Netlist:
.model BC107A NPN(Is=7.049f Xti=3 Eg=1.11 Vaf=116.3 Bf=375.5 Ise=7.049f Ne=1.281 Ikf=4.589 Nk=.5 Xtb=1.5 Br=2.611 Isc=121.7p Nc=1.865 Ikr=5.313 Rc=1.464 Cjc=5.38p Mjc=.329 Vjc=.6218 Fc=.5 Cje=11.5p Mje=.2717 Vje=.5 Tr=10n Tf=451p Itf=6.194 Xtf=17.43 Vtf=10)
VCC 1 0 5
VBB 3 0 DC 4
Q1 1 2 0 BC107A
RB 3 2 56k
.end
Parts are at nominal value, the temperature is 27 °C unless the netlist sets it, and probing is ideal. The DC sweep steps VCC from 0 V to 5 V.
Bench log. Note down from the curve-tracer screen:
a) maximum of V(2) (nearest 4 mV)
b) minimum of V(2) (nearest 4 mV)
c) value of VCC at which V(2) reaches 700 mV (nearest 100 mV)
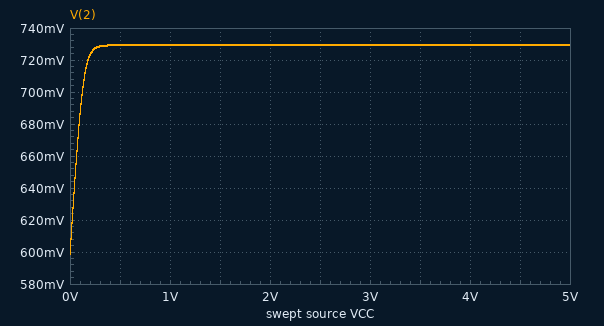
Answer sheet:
728 mV
600 mV
100 mV
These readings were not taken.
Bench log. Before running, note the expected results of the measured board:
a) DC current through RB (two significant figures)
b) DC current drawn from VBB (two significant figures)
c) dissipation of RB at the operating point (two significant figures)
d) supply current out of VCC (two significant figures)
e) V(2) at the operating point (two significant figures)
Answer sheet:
58 µA
58 µA
190 µW
13 mA
730 mV
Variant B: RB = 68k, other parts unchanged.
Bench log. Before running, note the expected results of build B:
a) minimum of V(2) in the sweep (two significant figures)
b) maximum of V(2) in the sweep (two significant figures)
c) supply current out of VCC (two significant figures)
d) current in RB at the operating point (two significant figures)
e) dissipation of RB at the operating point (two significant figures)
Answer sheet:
590 mV
720 mV
10 mA
48 µA
160 µW
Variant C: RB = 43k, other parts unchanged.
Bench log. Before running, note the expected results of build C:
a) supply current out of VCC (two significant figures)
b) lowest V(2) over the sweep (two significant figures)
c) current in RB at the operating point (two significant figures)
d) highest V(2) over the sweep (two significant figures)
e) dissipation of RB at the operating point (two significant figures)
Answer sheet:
17 mA
610 mV
76 µA
740 mV
250 µW
